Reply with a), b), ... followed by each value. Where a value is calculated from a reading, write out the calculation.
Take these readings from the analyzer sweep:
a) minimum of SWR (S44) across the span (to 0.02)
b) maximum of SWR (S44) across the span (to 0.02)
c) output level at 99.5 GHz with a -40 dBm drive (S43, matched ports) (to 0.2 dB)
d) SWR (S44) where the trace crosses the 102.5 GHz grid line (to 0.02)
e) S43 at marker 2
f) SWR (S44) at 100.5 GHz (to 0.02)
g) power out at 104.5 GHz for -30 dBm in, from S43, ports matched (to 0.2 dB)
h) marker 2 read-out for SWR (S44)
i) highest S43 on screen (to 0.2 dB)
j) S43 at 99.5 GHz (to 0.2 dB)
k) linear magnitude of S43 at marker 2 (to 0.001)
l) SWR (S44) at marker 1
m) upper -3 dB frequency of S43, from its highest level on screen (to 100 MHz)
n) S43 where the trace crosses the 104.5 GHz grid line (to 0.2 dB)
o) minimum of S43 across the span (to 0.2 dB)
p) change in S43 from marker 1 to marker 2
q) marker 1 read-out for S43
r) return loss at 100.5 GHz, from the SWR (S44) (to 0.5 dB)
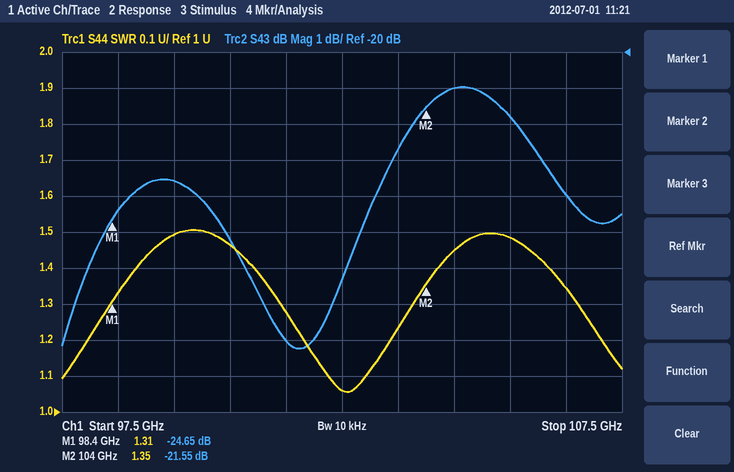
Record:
a) 1.06
b) 1.50
c) -40 dBm + (-23.6 dB) = -63.6 dBm
d) 1.06
e) -21.55 dB
f) 1.46
g) -30 dBm + (-21.0 dB) = -51.0 dBm
h) 1.35
i) -21.0 dB
j) -23.6 dB
k) 10^(-21.55/20) ≈ 0.084
l) 1.31
m) 106.5 GHz
n) -21.0 dB
o) -28.2 dB
p) -21.55 − (-24.65) = 3.10 dB
q) -24.65 dB
r) −20 log10((1.46 − 1)/(1.46 + 1)) ≈ 14.6 dB, so 14.5 dB to the nearest 0.5 dB
